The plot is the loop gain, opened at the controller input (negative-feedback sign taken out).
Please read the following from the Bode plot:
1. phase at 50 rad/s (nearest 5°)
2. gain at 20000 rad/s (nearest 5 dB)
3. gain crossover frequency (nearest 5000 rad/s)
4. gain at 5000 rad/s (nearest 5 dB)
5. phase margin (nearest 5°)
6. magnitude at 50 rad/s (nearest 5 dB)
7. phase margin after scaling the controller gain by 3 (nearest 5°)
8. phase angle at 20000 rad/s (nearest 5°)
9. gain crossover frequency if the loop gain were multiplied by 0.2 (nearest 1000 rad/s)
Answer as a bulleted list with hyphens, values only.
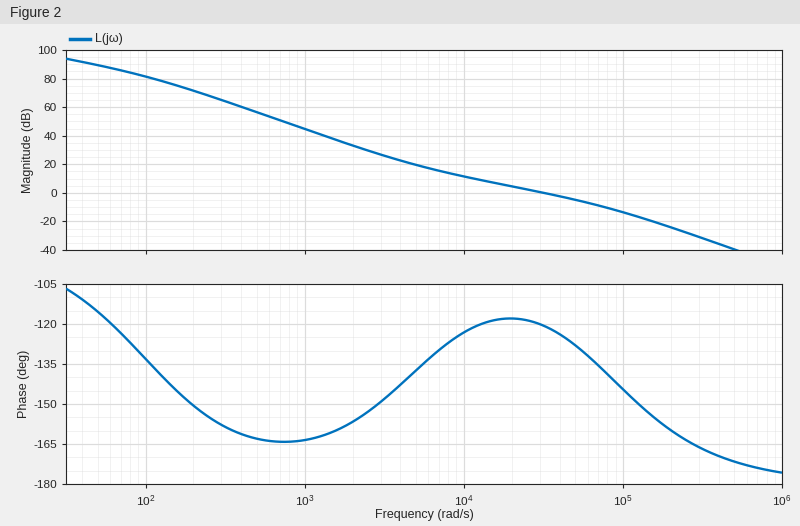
- -115°
- 5 dB
- 30000 rad/s
- 20 dB
- 60°
- 90 dB
- 45°
- -120°
- 8000 rad/s
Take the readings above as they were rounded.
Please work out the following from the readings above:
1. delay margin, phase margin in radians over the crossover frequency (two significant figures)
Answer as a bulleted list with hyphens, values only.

- 0.000035 s
